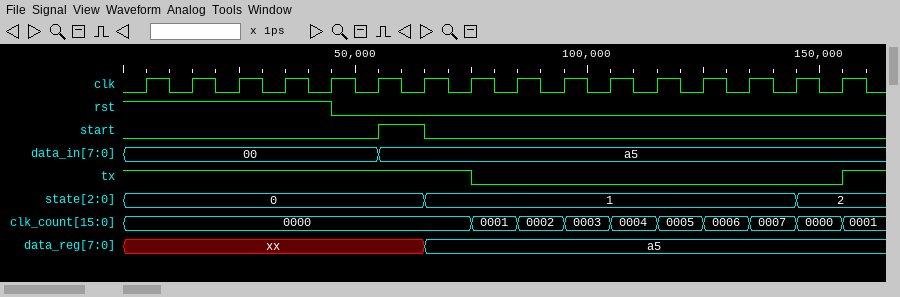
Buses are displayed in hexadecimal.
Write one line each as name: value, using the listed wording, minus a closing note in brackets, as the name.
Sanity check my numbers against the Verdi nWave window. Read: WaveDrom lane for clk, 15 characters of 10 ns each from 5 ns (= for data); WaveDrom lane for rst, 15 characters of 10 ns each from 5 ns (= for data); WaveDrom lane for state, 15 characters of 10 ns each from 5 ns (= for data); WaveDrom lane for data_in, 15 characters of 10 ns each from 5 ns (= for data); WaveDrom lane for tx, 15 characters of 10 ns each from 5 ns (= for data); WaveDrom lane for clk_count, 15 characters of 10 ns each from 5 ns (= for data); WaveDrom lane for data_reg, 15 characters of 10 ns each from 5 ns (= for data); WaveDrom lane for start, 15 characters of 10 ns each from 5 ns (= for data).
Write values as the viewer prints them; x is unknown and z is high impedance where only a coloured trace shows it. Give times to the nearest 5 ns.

WaveDrom lane for clk, 15 characters of 10 ns each from 5 ns: {name: 'clk', wave: 'p..............'}
WaveDrom lane for rst, 15 characters of 10 ns each from 5 ns: {name: 'rst', wave: '1...0..........'}
WaveDrom lane for state, 15 characters of 10 ns each from 5 ns: {name: 'state', wave: '=.....=.......=', data: '0 1 2'}
WaveDrom lane for data_in, 15 characters of 10 ns each from 5 ns: {name: 'data_in', wave: '=....=.........', data: '00 a5'}
WaveDrom lane for tx, 15 characters of 10 ns each from 5 ns: {name: 'tx', wave: '1......0.......'}
WaveDrom lane for clk_count, 15 characters of 10 ns each from 5 ns: {name: 'clk_count', wave: '=......========', data: '0000 0001 0002 0003 0004 0005 0006 0007 0000'}
WaveDrom lane for data_reg, 15 characters of 10 ns each from 5 ns: {name: 'data_reg', wave: 'x.....=........', data: 'a5'}
WaveDrom lane for start, 15 characters of 10 ns each from 5 ns: {name: 'start', wave: '0....10........'}
